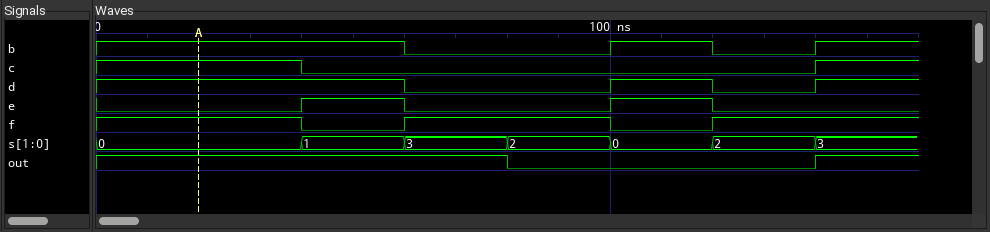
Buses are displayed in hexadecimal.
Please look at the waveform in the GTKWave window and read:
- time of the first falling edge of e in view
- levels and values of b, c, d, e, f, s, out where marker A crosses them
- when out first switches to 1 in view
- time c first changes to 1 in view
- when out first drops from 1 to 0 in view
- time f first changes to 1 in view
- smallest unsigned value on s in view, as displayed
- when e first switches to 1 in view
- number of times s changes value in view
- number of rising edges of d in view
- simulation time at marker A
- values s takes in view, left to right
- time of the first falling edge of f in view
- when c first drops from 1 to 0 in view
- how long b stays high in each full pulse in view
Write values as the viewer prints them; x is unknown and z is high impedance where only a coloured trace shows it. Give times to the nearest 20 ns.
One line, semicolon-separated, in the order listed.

60 ns; b=1, c=1, d=1, e=0, f=1, s=0, out=1; 140 ns; 140 ns; 80 ns; 60 ns; 0; 40 ns; 6; 2; 20 ns; 0, 1, 3, 2, 0, 2, 3; 40 ns; 40 ns; 20 ns
